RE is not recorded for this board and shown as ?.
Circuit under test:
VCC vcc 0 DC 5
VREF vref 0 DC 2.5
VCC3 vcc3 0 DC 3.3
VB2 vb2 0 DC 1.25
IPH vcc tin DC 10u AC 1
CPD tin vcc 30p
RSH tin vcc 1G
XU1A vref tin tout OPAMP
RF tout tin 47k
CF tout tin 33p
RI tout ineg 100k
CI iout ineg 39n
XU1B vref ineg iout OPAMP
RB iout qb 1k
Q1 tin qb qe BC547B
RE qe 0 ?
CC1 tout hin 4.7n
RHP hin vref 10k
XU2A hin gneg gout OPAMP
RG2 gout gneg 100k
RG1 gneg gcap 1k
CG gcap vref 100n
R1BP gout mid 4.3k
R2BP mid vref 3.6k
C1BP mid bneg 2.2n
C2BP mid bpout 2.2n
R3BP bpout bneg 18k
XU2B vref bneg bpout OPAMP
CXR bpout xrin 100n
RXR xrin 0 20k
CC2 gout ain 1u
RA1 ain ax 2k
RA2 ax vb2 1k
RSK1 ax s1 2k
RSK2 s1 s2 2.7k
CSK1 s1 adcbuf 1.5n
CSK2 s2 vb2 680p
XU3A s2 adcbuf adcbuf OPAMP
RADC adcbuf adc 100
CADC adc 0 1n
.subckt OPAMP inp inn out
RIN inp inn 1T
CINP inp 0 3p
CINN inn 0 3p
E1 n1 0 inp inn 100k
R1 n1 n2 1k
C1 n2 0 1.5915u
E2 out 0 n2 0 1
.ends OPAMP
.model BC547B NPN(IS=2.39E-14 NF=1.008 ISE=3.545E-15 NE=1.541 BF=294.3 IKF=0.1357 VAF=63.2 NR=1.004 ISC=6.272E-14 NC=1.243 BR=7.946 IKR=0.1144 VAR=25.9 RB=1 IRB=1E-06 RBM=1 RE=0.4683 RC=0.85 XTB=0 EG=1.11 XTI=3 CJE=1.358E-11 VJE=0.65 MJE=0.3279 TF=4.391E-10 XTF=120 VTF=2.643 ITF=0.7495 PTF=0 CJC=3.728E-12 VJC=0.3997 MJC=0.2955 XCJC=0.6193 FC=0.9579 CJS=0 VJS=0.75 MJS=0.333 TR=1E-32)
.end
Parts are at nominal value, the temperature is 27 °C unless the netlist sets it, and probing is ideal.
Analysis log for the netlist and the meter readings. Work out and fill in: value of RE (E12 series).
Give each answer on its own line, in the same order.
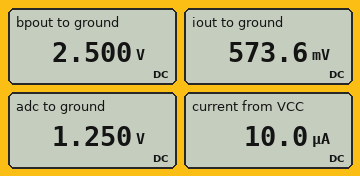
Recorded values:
5.6 kΩ
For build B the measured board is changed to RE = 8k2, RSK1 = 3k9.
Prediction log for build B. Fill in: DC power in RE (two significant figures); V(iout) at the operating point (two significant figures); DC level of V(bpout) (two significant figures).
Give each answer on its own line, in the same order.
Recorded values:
830 nW
600 mV
2.5 V
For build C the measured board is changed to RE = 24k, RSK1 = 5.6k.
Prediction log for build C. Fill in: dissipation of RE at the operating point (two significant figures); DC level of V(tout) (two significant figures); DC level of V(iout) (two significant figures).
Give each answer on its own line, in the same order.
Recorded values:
2.4 µW
2.5 V
760 mV
